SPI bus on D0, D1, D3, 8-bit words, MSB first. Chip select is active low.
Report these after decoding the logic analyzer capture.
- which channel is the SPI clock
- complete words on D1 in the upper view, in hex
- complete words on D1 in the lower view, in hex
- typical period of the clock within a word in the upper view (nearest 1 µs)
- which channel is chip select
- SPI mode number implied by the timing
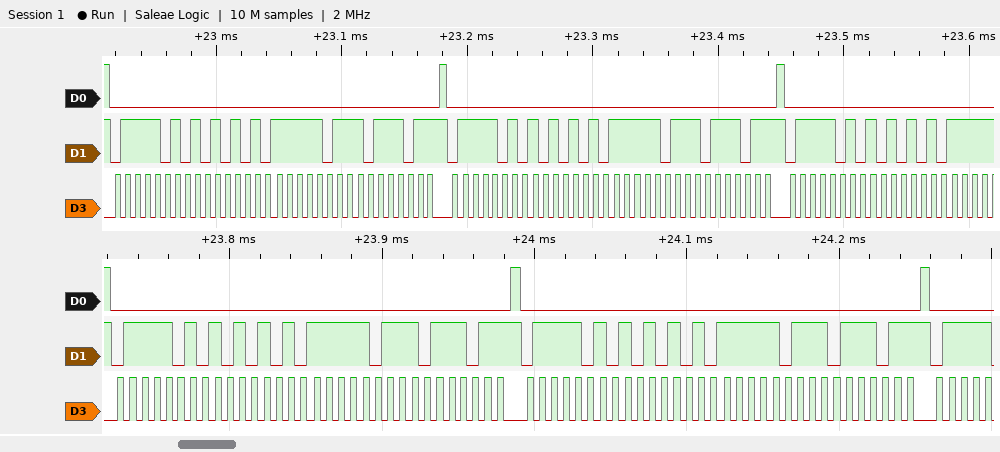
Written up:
D3
7A, AA, FB, BB, 7A, AA, FB, BB, 7A, AA
7A, AA, FB, BB, 7A, AA, FB, BB
8 µs
D0
0
